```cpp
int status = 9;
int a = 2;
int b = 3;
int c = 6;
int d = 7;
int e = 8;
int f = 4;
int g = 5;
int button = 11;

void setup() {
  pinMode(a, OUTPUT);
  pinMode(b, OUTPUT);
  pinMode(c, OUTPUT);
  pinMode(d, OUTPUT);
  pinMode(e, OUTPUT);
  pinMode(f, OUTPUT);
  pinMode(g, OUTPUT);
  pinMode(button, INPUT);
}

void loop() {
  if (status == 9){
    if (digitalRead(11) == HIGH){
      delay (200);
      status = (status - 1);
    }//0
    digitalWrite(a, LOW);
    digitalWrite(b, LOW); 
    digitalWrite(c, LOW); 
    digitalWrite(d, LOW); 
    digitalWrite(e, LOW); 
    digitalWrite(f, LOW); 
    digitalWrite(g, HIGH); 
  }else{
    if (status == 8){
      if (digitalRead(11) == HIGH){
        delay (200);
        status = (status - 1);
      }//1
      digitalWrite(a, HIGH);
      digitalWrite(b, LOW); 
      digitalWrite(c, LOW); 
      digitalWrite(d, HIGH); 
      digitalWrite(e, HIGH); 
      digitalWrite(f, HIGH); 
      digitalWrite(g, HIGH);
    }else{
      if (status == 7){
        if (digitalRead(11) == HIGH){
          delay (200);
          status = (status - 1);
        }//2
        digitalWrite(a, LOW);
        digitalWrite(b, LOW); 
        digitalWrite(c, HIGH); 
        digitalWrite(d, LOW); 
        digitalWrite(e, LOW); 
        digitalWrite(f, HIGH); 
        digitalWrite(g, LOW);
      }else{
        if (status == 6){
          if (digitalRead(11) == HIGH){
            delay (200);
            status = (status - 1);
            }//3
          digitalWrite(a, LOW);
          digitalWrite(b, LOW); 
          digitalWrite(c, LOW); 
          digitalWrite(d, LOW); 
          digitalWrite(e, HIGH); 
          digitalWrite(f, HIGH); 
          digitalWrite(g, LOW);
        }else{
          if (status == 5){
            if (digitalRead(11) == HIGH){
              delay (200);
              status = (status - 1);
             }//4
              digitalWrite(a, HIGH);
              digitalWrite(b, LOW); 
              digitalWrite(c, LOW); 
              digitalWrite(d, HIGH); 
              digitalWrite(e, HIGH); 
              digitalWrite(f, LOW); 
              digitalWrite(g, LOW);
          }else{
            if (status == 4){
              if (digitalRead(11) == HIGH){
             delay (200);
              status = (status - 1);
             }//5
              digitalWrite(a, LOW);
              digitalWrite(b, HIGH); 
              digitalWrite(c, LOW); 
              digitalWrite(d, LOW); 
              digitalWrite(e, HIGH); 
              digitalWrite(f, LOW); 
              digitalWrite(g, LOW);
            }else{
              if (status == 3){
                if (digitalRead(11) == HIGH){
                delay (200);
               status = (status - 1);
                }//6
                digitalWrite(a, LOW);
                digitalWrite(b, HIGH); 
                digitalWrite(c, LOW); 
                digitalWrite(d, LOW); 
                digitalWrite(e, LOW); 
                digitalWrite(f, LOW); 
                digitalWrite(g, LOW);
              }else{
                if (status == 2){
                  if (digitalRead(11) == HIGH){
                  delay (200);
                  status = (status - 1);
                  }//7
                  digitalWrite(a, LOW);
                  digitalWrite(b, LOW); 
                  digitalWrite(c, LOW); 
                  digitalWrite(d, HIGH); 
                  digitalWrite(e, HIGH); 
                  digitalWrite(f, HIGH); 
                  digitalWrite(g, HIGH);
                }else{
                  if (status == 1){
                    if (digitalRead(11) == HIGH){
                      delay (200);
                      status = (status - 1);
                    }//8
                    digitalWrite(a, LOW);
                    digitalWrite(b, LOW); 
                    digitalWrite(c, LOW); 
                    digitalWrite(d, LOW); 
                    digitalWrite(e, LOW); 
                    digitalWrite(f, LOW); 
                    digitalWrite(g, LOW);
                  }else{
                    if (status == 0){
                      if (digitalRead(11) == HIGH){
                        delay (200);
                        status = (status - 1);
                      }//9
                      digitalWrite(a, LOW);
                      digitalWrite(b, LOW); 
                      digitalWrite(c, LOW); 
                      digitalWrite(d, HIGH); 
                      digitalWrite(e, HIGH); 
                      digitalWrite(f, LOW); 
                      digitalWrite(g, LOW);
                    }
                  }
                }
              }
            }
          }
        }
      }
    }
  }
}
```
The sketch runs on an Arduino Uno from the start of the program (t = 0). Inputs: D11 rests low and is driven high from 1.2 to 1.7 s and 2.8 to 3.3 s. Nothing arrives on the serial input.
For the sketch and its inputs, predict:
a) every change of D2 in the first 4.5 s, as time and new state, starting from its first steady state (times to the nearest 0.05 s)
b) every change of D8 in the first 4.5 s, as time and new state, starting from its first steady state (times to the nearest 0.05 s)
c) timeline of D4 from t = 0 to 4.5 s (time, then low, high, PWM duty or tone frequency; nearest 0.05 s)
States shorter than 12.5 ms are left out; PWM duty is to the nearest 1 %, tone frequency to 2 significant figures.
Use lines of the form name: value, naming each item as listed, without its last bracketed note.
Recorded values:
every change of D2 in the first 4.5 s, as time and new state, starting from its first steady state: 0 s low; 1.6 s high; 1.8 s low; 3.2 s high; 3.4 s low
every change of D8 in the first 4.5 s, as time and new state, starting from its first steady state: 0 s low; 1.6 s high; 3.4 s low
timeline of D4 from t = 0 to 4.5 s: 0 s low; 1.6 s high; 3.2 s low
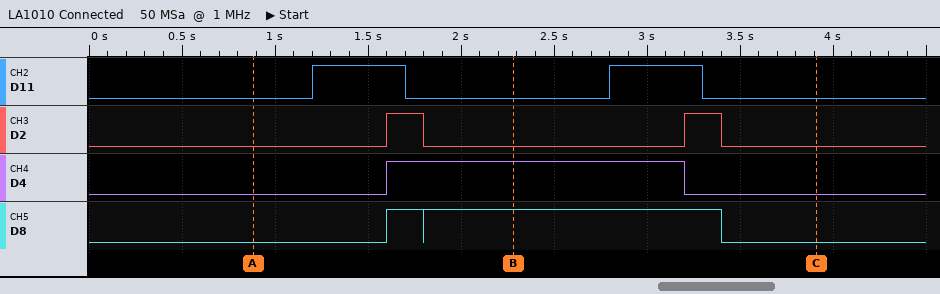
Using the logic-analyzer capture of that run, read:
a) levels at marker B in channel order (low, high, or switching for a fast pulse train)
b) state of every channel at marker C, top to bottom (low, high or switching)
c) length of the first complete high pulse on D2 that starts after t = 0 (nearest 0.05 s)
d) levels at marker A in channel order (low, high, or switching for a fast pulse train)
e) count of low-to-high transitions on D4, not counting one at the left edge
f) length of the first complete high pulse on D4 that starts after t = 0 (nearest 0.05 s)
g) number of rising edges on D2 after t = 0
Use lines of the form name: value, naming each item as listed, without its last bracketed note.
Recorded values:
levels at marker B in channel order: D11 low, D2 low, D4 high, D8 high
state of every channel at marker C, top to bottom: D11 low, D2 low, D4 low, D8 low
length of the first complete high pulse on D2 that starts after t = 0: 0.20 s
levels at marker A in channel order: D11 low, D2 low, D4 low, D8 low
count of low-to-high transitions on D4, not counting one at the left edge: 1
length of the first complete high pulse on D4 that starts after t = 0: 1.60 s
number of rising edges on D2 after t = 0: 2
